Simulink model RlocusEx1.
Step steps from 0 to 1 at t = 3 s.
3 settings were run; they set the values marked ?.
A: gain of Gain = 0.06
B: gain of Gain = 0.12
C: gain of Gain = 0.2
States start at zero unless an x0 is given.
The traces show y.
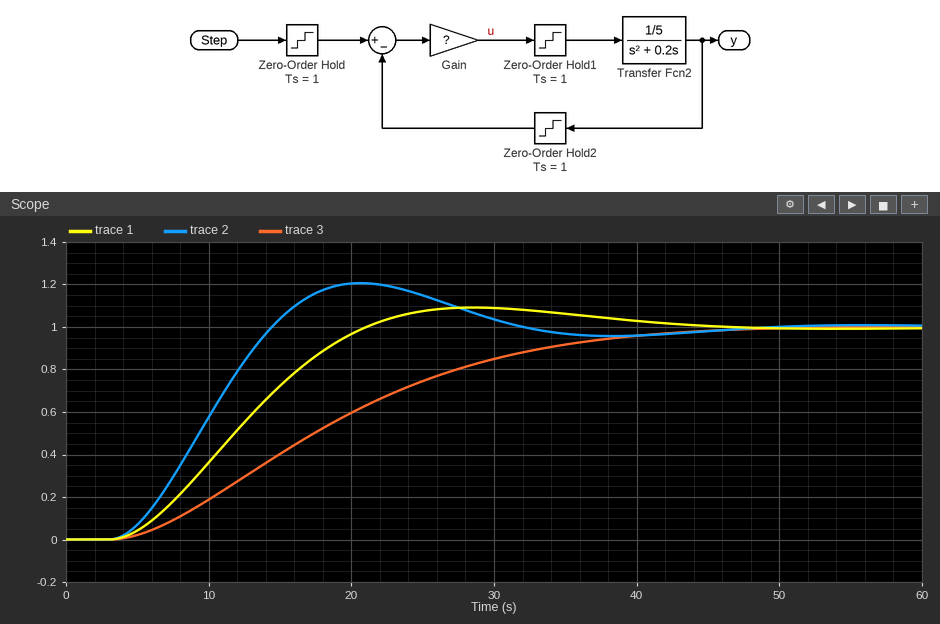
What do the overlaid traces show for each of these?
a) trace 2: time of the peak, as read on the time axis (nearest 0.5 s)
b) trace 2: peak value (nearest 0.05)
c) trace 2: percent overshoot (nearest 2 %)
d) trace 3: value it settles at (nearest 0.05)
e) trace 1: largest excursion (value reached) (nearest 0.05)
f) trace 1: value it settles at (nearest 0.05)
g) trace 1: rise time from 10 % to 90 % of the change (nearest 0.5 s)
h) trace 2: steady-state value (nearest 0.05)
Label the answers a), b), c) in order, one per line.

a) 20.5 s
b) 1.20
c) 20 %
d) 1.00
e) 1.10
f) 1.00
g) 12.0 s
h) 1.00
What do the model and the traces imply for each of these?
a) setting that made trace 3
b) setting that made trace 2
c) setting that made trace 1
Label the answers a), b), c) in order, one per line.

a) A
b) C
c) B
